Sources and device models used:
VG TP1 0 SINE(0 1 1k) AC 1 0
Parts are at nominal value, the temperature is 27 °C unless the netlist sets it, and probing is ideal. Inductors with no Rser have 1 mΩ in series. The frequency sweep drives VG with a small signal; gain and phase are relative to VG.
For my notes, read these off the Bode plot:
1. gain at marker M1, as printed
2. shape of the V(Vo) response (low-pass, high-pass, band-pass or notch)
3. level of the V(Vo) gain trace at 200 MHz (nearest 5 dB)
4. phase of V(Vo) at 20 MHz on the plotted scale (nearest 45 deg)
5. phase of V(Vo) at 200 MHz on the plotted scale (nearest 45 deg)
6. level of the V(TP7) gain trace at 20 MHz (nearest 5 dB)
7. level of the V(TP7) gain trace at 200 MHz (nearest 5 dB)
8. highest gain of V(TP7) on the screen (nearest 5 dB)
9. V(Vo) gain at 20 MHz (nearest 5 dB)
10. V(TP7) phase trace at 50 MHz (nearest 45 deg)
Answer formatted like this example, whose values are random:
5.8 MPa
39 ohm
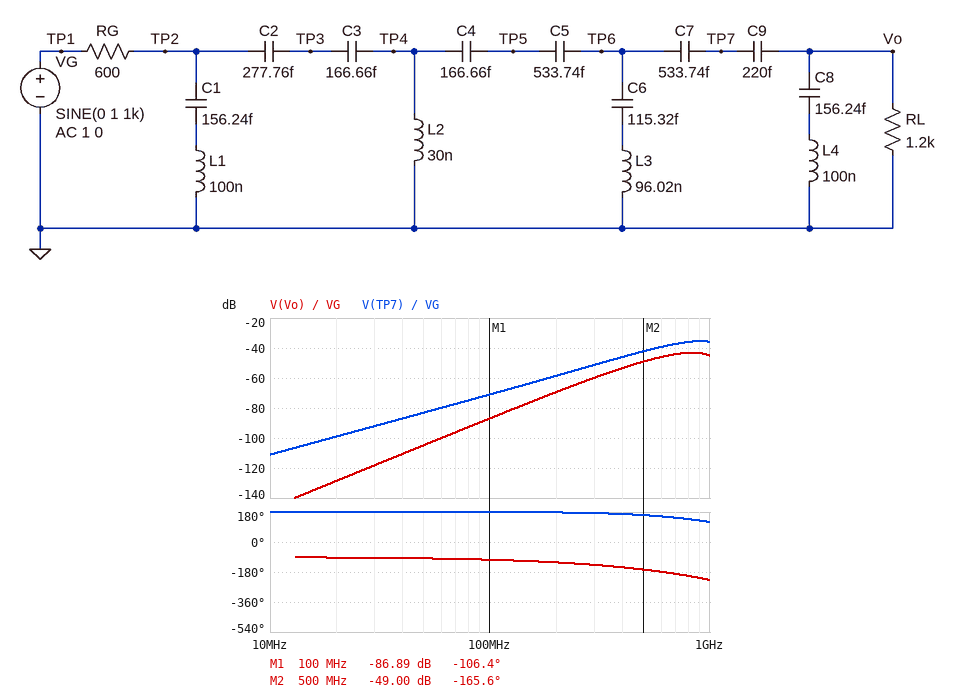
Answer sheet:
-86.89 dB
high-pass
-70 dB
-90 deg
-135 deg
-100 dB
-60 dB
-35 dB
-130 dB
180 deg
